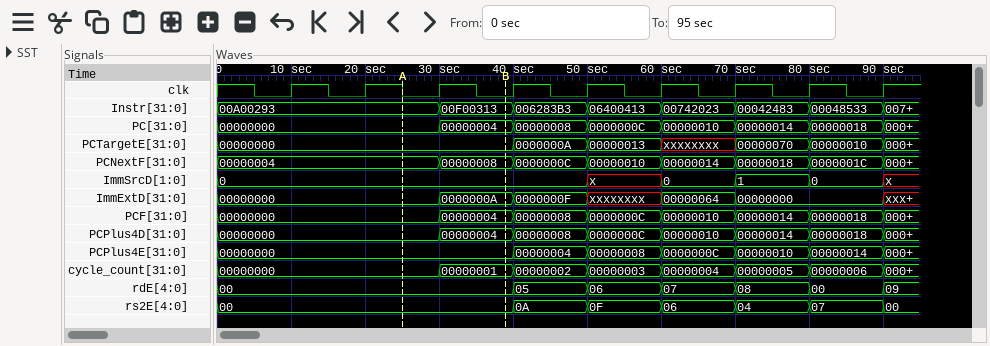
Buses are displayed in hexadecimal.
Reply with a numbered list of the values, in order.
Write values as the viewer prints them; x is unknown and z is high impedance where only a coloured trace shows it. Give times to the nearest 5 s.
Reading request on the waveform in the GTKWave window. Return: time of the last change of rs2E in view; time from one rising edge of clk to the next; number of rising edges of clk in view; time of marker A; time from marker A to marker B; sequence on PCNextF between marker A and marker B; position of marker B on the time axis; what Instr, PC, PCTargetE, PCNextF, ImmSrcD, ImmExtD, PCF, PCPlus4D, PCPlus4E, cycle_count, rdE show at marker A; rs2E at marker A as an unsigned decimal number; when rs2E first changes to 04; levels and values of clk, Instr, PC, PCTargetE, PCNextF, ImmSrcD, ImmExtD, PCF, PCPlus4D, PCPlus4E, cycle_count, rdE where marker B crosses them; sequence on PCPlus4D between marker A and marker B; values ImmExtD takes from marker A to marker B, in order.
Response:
1. 90 s
2. 10 s
3. 9
4. 25 s
5. 15 s
6. 00000004, 00000008
7. 40 s
8. Instr=00A00293, PC=00000000, PCTargetE=00000000, PCNextF=00000004, ImmSrcD=0, ImmExtD=00000000, PCF=00000000, PCPlus4D=00000000, PCPlus4E=00000000, cycle_count=00000000, rdE=00
9. 0
10. 70 s
11. clk=0, Instr=00F00313, PC=00000004, PCTargetE=00000000, PCNextF=00000008, ImmSrcD=0, ImmExtD=0000000A, PCF=00000004, PCPlus4D=00000004, PCPlus4E=00000000, cycle_count=00000001, rdE=00
12. 00000000, 00000004
13. 00000000, 0000000A
